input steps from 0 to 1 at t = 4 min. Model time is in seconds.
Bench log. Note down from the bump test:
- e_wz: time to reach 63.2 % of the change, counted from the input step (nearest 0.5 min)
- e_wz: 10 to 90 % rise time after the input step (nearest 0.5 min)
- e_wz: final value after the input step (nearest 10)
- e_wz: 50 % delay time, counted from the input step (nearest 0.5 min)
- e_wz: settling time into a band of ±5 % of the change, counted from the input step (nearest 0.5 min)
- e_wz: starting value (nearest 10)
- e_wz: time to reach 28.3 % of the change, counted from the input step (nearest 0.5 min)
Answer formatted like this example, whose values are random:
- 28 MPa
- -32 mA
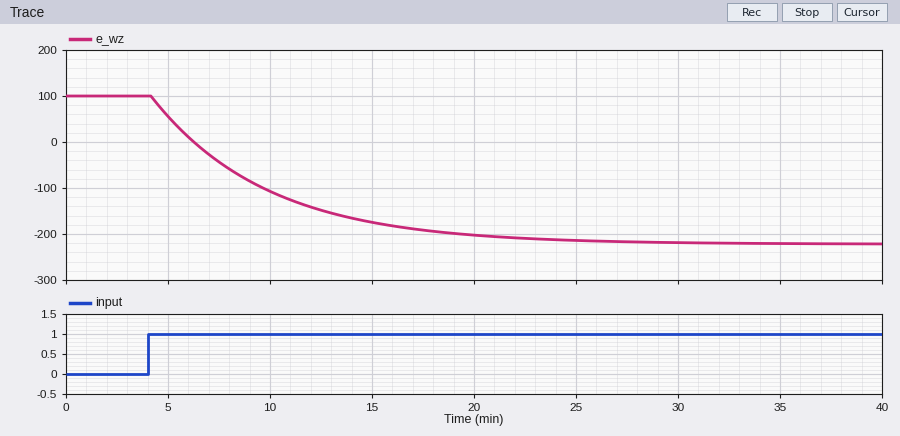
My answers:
- 6.0 min
- 12.5 min
- -220
- 4.0 min
- 17.0 min
- 100
- 2.0 min
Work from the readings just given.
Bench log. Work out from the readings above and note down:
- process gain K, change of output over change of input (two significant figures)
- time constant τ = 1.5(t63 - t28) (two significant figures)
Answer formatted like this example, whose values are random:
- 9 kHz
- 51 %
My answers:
- -320
- 6.0 min
